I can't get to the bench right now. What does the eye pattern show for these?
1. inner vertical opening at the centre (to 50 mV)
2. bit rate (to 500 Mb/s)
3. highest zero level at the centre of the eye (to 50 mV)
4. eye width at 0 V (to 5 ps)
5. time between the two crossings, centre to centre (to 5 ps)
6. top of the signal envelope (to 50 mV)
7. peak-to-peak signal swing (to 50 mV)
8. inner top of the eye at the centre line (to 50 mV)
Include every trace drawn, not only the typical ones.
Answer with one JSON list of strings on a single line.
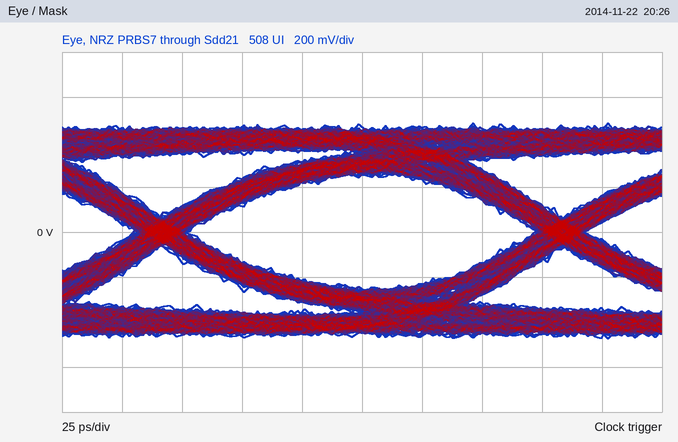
["500 mV", "6.0 Gb/s", "-250 mV", "145 ps", "165 ps", "500 mV", "950 mV", "250 mV"]
